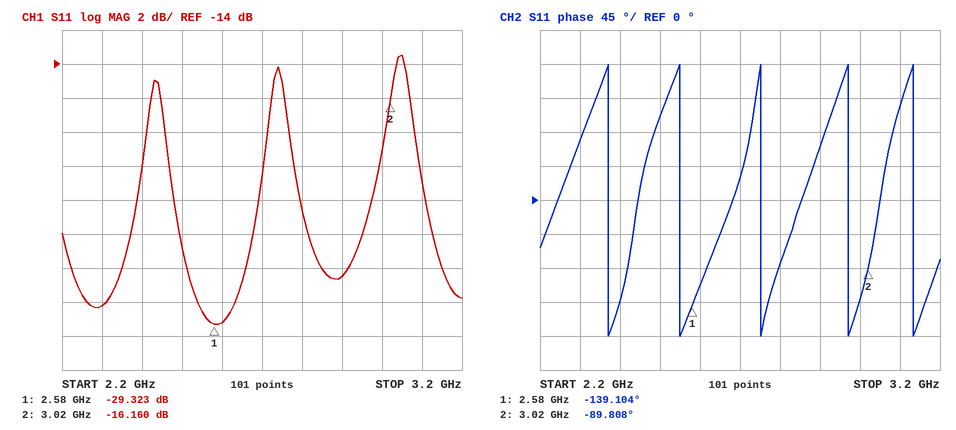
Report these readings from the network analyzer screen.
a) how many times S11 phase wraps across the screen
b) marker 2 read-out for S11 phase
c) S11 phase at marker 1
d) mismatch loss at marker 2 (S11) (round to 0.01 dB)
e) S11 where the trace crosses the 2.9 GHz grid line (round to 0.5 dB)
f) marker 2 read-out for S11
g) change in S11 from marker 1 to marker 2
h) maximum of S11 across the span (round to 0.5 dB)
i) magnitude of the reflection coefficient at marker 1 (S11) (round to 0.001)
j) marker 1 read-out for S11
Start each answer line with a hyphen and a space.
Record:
- 5
- -89.808°
- -139.104°
- 0.11 dB
- -26.5 dB
- -16.160 dB
- 13.163 dB
- -13.5 dB
- 0.034
- -29.323 dB
